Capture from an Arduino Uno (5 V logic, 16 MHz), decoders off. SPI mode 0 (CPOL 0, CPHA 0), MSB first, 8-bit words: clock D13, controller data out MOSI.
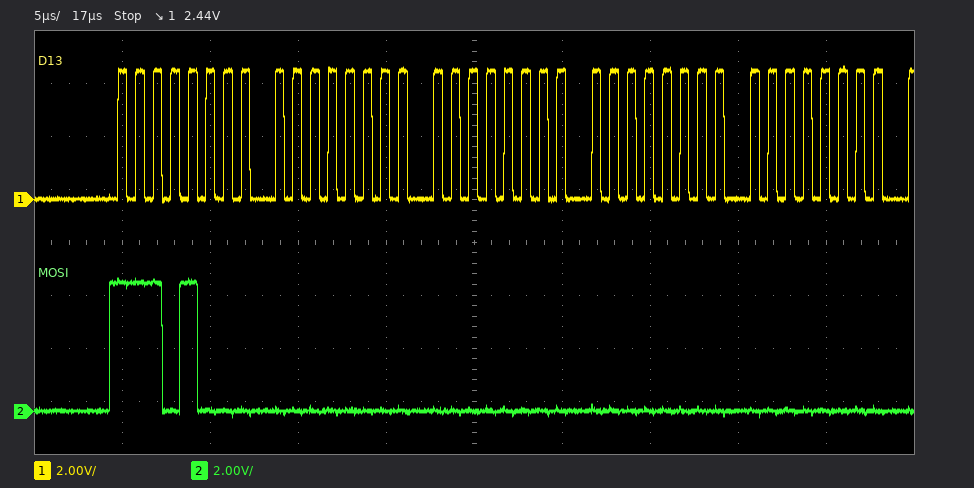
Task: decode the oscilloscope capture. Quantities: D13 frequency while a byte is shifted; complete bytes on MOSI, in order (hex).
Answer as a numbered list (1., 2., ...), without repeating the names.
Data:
1. 1 MHz
2. E8 00 00 00 00
